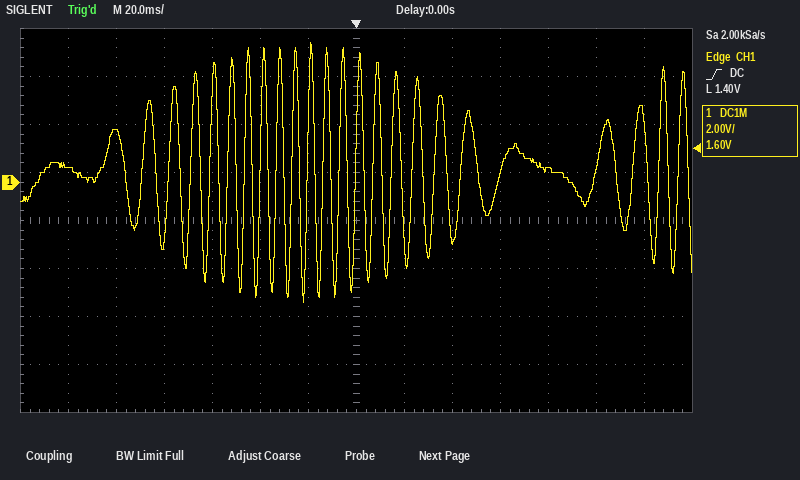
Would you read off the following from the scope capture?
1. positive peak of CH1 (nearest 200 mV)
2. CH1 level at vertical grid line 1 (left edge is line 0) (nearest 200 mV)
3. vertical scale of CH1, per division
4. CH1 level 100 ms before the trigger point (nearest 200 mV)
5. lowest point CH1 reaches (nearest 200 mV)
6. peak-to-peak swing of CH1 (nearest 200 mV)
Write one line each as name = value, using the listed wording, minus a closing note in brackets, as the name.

positive peak of CH1 = 5.8 V
CH1 level at vertical grid line 1 (left edge is line 0) = 600 mV
vertical scale of CH1, per division = 2 V
CH1 level 100 ms before the trigger point = 2.2 V
lowest point CH1 reaches = -5.0 V
peak-to-peak swing of CH1 = 10.8 V
